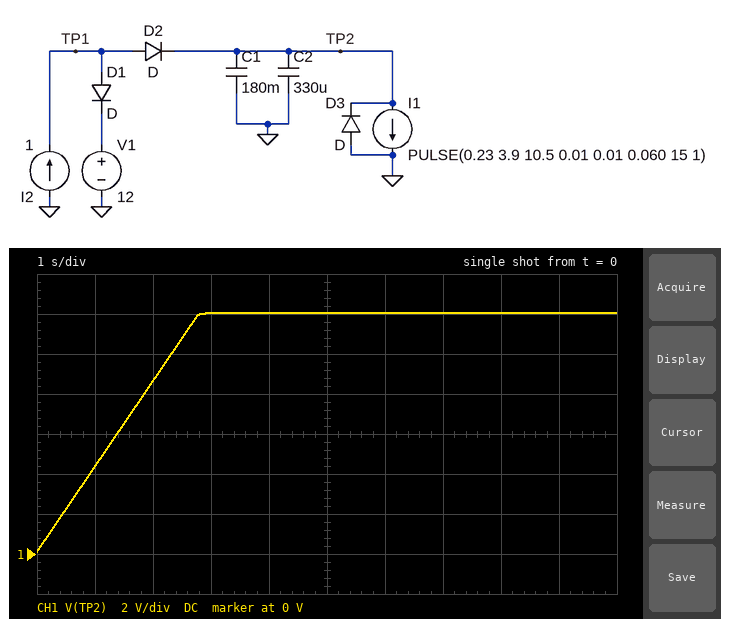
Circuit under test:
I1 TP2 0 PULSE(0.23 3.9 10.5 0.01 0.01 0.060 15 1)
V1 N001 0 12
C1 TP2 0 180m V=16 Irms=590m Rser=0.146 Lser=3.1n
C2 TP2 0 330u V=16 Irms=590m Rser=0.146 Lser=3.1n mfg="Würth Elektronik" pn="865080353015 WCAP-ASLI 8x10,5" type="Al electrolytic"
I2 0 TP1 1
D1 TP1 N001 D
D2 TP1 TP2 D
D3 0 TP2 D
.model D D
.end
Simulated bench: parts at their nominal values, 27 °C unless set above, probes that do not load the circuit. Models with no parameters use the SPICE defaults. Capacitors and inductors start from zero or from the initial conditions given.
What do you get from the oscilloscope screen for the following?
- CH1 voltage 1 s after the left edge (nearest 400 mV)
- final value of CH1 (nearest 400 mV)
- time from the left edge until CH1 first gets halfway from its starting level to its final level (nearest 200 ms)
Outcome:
4.4 V
12.0 V
1.4 s
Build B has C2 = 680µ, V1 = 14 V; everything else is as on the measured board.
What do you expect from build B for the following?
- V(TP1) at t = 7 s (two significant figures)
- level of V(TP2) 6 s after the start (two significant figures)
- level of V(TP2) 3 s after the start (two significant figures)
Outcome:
15 V
14 V
13 V
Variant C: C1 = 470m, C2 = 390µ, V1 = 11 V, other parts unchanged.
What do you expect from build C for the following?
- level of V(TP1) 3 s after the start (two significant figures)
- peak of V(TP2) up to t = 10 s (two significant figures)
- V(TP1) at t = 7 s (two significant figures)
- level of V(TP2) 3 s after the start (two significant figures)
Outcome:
5.9 V
11 V
12 V
5.0 V
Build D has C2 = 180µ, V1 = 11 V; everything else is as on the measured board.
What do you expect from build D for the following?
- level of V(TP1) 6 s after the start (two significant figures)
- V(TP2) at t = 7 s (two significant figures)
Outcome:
12 V
11 V
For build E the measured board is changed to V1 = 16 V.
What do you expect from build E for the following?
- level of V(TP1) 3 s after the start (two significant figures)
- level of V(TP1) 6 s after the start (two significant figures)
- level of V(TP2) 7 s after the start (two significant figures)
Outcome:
14 V
17 V
16 V
